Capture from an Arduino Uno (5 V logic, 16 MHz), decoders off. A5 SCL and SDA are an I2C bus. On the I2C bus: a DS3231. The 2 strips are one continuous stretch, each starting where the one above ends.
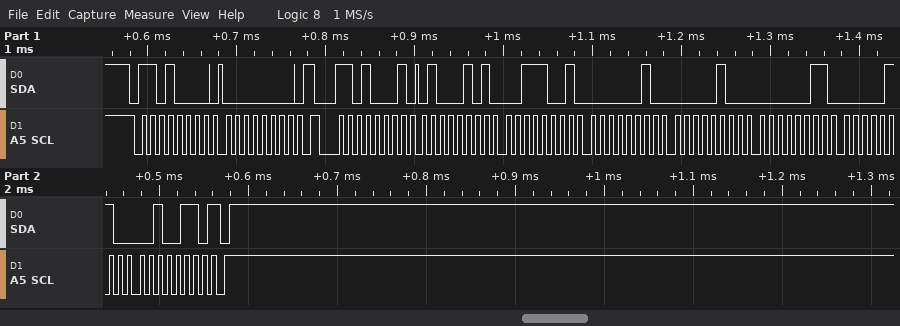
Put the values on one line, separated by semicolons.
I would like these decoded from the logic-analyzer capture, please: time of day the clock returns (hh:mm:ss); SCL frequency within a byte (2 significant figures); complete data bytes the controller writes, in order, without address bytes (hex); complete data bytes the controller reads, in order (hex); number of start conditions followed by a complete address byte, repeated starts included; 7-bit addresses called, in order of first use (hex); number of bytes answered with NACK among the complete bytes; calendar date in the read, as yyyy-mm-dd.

02:39:45; 100 kHz; 00; 45 39 02 04 03 06 26; 2; 0x68; 1; 2026-06-03
